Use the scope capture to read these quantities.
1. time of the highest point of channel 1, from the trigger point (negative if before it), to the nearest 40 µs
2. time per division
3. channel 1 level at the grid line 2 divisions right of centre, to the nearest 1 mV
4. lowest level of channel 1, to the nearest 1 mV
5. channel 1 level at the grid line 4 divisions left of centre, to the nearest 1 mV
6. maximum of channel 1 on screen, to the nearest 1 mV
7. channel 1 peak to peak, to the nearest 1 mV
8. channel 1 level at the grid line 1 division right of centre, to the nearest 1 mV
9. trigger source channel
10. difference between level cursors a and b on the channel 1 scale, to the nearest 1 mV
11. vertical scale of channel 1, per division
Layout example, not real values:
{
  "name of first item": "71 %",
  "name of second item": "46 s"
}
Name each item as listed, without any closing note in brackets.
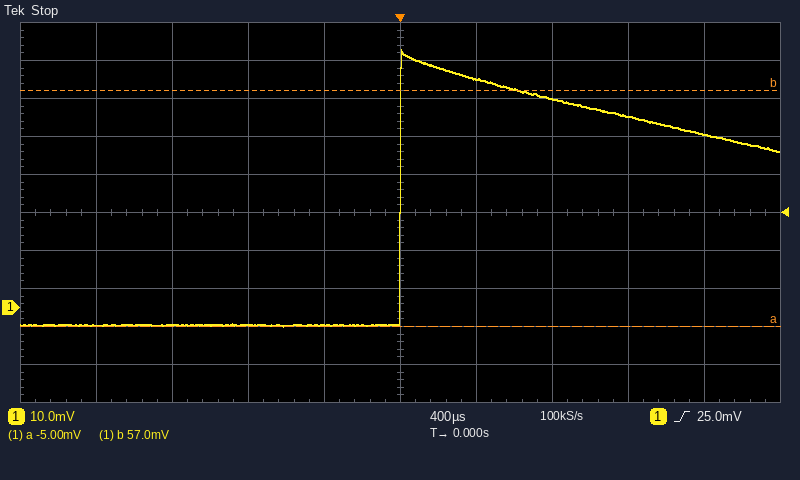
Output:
{
  "time of the highest point of channel 1, from the trigger point (negative if before it), to the nearest 40 µs": "0 µs",
  "time per division": "400 µs",
  "channel 1 level at the grid line 2 divisions right of centre, to the nearest 1 mV": "55 mV",
  "lowest level of channel 1, to the nearest 1 mV": "-5 mV",
  "channel 1 level at the grid line 4 divisions left of centre, to the nearest 1 mV": "-5 mV",
  "maximum of channel 1 on screen, to the nearest 1 mV": "68 mV",
  "channel 1 peak to peak, to the nearest 1 mV": "73 mV",
  "channel 1 level at the grid line 1 division right of centre, to the nearest 1 mV": "60 mV",
  "trigger source channel": "channel 1",
  "difference between level cursors a and b on the channel 1 scale, to the nearest 1 mV": "62 mV",
  "vertical scale of channel 1, per division": "10 mV"
}
